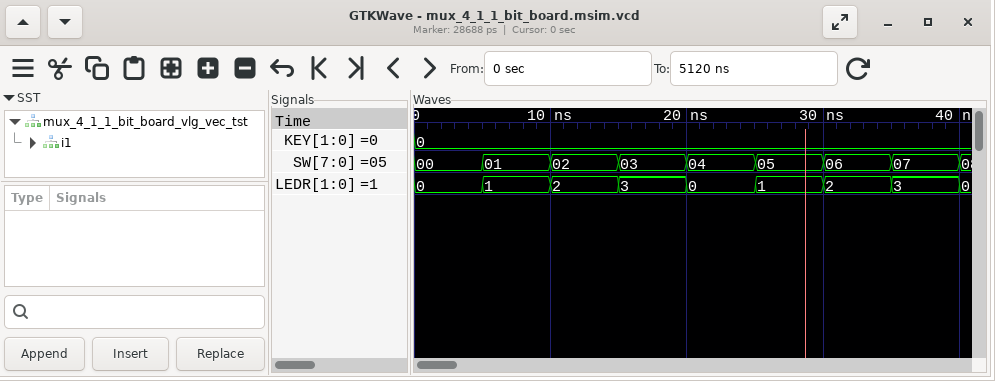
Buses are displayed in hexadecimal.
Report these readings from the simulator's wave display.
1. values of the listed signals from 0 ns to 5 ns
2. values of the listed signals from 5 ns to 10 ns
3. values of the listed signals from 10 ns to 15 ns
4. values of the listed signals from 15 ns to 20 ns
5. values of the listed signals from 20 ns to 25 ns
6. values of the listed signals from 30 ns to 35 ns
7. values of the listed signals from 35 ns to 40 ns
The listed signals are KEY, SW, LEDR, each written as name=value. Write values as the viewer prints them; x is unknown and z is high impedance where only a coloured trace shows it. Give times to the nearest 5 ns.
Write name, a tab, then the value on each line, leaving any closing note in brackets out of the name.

values of the listed signals from 0 ns to 5 ns	KEY=0, SW=00, LEDR=0
values of the listed signals from 5 ns to 10 ns	KEY=0, SW=01, LEDR=1
values of the listed signals from 10 ns to 15 ns	KEY=0, SW=02, LEDR=2
values of the listed signals from 15 ns to 20 ns	KEY=0, SW=03, LEDR=3
values of the listed signals from 20 ns to 25 ns	KEY=0, SW=04, LEDR=0
values of the listed signals from 30 ns to 35 ns	KEY=0, SW=06, LEDR=2
values of the listed signals from 35 ns to 40 ns	KEY=0, SW=07, LEDR=3
